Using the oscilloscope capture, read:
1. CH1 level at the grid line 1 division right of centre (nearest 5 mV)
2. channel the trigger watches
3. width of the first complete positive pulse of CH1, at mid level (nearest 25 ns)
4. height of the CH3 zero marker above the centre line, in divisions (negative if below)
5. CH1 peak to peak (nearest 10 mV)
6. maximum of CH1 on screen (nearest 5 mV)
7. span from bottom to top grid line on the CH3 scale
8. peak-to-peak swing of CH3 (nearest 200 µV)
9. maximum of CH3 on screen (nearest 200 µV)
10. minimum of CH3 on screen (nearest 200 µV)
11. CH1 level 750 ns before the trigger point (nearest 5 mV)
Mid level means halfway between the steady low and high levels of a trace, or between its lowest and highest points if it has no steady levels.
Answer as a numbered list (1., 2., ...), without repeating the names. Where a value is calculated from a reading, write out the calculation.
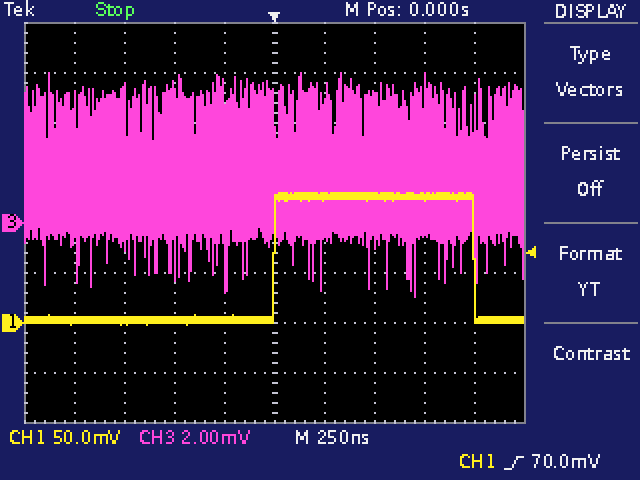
1. 125 mV
2. CH1
3. 1.000 µs
4. 0.0 div
5. 130 mV
6. 130 mV
7. 16 mV
8. 6.0 mV − (-3.0 mV) = 9.0 mV
9. 6.0 mV
10. -3.0 mV
11. 0 mV
